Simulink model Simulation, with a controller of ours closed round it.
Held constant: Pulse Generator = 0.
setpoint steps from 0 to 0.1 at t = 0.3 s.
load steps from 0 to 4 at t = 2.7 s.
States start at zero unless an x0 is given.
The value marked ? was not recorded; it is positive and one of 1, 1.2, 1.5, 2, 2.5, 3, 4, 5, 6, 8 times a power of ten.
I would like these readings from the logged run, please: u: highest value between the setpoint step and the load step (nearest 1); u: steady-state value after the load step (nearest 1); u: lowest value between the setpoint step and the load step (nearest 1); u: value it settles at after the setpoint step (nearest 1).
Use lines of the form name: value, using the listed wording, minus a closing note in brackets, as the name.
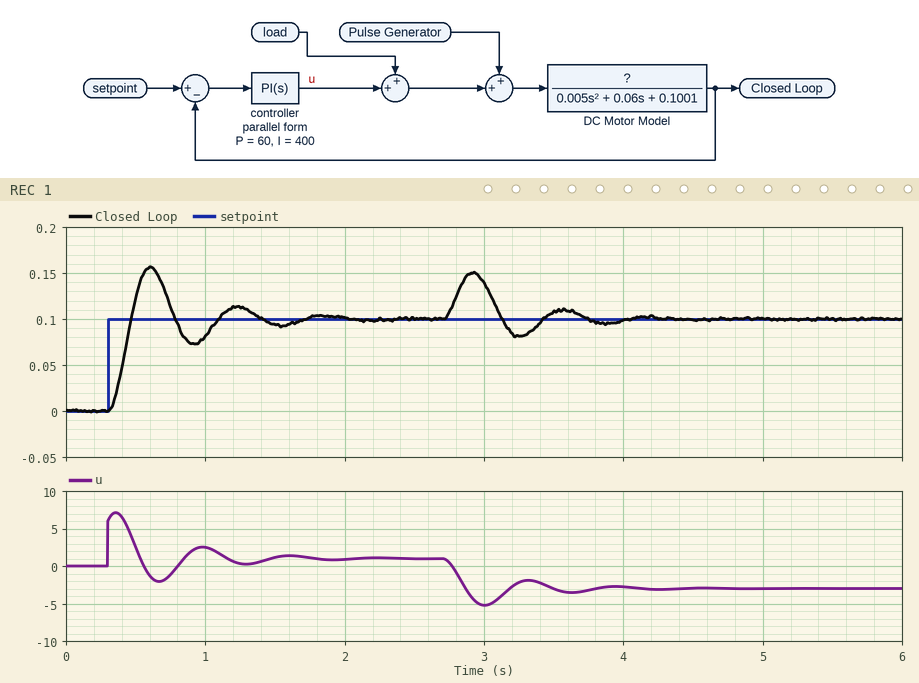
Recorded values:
u: highest value between the setpoint step and the load step: 7
u: steady-state value after the load step: -3
u: lowest value between the setpoint step and the load step: -2
u: value it settles at after the setpoint step: 1
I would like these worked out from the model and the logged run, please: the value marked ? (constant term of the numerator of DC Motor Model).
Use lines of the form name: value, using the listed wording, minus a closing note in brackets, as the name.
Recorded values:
the value marked ?: 0.01
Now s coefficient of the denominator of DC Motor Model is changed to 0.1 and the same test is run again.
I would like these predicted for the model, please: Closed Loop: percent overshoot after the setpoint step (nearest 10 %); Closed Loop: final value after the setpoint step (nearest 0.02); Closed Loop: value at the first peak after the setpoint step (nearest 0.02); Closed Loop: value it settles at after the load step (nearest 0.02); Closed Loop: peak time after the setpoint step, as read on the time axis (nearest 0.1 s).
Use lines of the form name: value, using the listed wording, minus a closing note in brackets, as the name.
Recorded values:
Closed Loop: percent overshoot after the setpoint step: 40 %
Closed Loop: final value after the setpoint step: 0.10
Closed Loop: value at the first peak after the setpoint step: 0.14
Closed Loop: value it settles at after the load step: 0.10
Closed Loop: peak time after the setpoint step, as read on the time axis: 0.7 s
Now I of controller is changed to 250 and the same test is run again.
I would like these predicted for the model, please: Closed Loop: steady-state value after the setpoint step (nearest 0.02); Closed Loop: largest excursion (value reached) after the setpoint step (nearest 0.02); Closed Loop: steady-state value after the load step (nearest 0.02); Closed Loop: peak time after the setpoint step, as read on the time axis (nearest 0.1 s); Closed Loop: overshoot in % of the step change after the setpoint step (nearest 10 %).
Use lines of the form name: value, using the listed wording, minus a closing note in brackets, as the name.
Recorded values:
Closed Loop: steady-state value after the setpoint step: 0.10
Closed Loop: largest excursion (value reached) after the setpoint step: 0.14
Closed Loop: steady-state value after the load step: 0.10
Closed Loop: peak time after the setpoint step, as read on the time axis: 0.6 s
Closed Loop: overshoot in % of the step change after the setpoint step: 40 %
